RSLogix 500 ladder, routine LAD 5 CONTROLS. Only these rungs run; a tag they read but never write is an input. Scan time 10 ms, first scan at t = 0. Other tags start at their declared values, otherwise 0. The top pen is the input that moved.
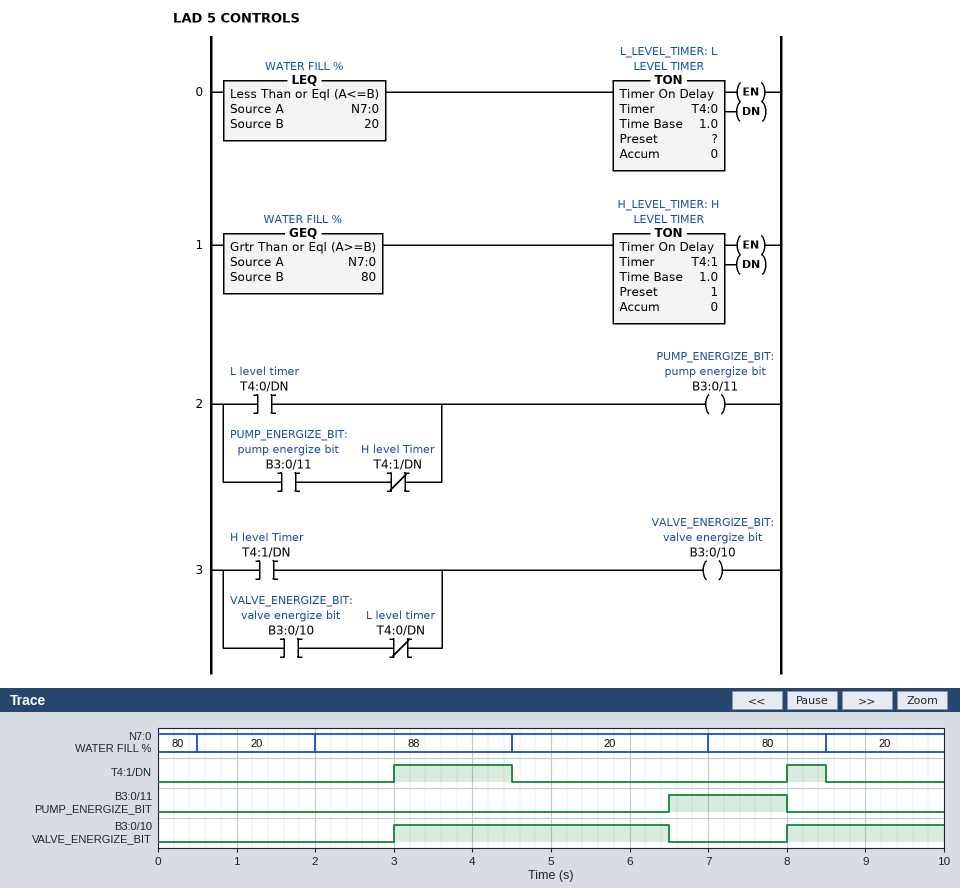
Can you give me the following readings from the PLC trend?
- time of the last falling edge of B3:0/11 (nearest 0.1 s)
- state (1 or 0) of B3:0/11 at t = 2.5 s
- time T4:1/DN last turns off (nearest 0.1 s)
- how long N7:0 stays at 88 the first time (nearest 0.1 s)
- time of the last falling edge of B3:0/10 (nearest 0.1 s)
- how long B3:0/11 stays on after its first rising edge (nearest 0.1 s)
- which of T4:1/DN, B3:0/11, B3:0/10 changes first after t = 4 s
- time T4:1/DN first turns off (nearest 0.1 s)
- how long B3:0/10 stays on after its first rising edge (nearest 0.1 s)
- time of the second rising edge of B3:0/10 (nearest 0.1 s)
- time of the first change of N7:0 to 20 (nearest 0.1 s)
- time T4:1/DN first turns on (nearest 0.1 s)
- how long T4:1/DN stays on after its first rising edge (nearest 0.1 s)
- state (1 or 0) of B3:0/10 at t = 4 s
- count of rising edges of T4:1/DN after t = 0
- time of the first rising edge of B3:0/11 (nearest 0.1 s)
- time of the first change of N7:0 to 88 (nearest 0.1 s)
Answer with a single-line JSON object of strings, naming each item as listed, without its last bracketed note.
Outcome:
{"time of the last falling edge of B3:0/11": "8.0 s", "state (1 or 0) of B3:0/11 at t = 2.5 s": "0", "time T4:1/DN last turns off": "8.5 s", "how long N7:0 stays at 88 the first time": "2.5 s", "time of the last falling edge of B3:0/10": "6.5 s", "how long B3:0/11 stays on after its first rising edge": "1.5 s", "which of T4:1/DN, B3:0/11, B3:0/10 changes first after t = 4 s": "T4:1/DN", "time T4:1/DN first turns off": "4.5 s", "how long B3:0/10 stays on after its first rising edge": "3.5 s", "time of the second rising edge of B3:0/10": "8.0 s", "time of the first change of N7:0 to 20": "0.5 s", "time T4:1/DN first turns on": "3.0 s", "how long T4:1/DN stays on after its first rising edge": "1.5 s", "state (1 or 0) of B3:0/10 at t = 4 s": "1", "count of rising edges of T4:1/DN after t = 0": "2", "time of the first rising edge of B3:0/11": "6.5 s", "time of the first change of N7:0 to 88": "2.0 s"}
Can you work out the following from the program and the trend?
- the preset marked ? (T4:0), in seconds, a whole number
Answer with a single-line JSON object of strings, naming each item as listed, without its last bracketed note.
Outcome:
{"the preset marked ? (T4:0), in seconds, a whole number": "2 s"}
